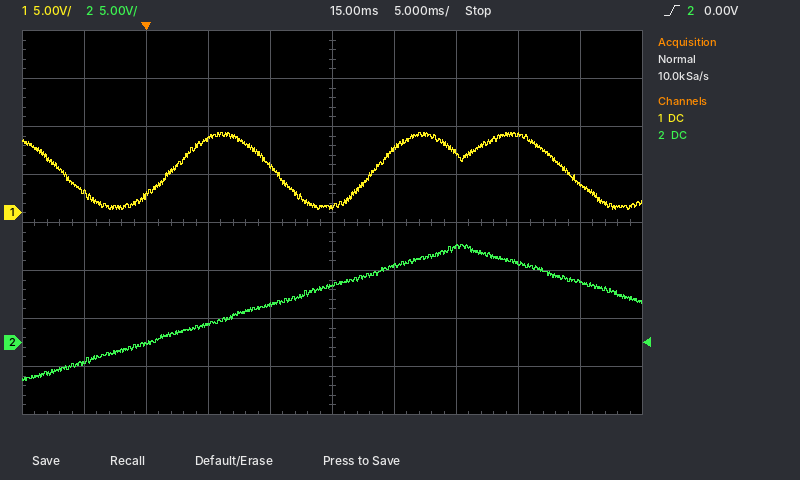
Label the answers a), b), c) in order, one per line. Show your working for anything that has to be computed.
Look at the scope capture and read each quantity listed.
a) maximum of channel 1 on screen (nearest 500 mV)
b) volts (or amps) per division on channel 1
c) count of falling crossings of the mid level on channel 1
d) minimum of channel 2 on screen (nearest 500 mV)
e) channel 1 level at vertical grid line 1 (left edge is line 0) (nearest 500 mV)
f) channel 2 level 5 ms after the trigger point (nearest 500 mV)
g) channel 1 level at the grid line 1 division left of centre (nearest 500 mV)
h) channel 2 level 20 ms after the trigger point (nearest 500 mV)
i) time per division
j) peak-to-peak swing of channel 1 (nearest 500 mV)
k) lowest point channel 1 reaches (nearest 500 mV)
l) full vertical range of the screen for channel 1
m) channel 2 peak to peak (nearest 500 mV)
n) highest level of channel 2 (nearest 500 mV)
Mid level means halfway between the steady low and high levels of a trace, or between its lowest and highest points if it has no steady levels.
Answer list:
a) 8.5 V
b) 5 V
c) 3
d) -4.0 V
e) 2.0 V
f) 2.0 V
g) 5.0 V
h) 8.0 V
i) 5 ms
j) 8.5 V − (500 mV) = 8.0 V
k) 500 mV
l) 40 V
m) 10.0 V − (-4.0 V) = 14.0 V
n) 10.0 V
